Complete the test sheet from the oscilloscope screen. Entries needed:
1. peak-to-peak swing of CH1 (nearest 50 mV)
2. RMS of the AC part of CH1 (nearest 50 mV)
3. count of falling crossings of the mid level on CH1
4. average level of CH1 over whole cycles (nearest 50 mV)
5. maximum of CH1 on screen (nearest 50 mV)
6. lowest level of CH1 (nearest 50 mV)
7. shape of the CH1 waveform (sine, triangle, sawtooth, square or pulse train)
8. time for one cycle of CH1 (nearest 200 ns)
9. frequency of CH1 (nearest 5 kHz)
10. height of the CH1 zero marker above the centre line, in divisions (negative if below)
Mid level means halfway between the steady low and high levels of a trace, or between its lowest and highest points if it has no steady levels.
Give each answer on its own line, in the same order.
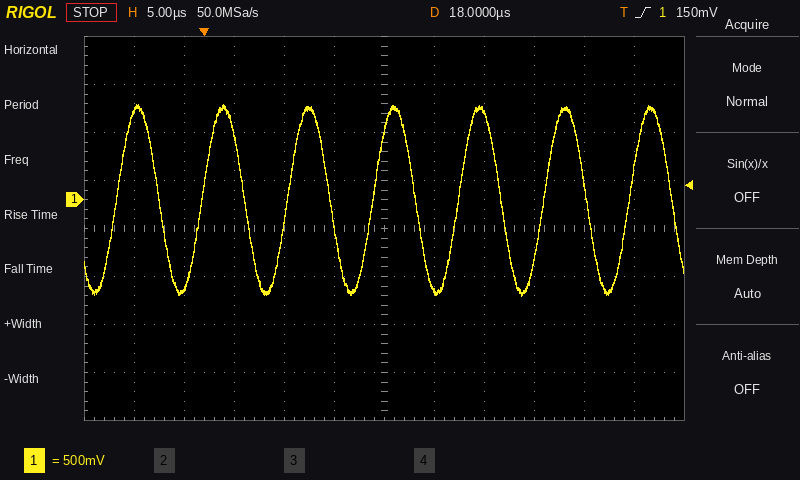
2.00 V
700 mV
7
0 mV
1.00 V
-1.00 V
sine
8.6 µs
115 kHz
+0.6 div
